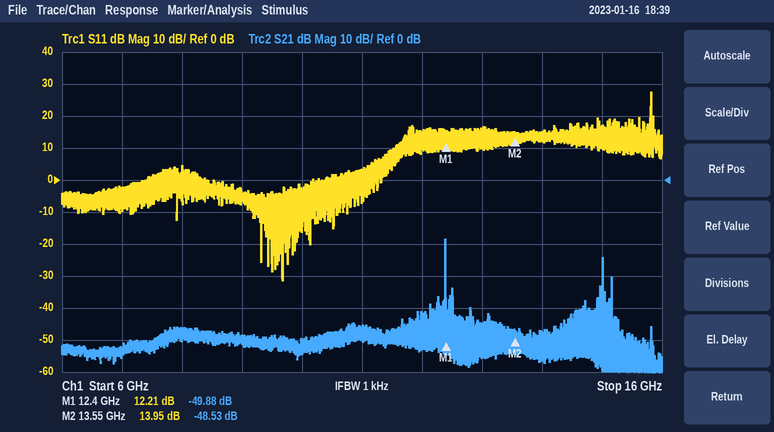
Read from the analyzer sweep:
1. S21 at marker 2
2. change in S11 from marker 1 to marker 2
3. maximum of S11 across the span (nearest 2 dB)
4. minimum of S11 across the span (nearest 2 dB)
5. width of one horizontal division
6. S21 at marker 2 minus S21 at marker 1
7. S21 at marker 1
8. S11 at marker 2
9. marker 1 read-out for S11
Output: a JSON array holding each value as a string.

["-48.53 dB", "1.74 dB", "28 dB", "-32 dB", "1 GHz", "1.35 dB", "-49.88 dB", "13.95 dB", "12.21 dB"]
